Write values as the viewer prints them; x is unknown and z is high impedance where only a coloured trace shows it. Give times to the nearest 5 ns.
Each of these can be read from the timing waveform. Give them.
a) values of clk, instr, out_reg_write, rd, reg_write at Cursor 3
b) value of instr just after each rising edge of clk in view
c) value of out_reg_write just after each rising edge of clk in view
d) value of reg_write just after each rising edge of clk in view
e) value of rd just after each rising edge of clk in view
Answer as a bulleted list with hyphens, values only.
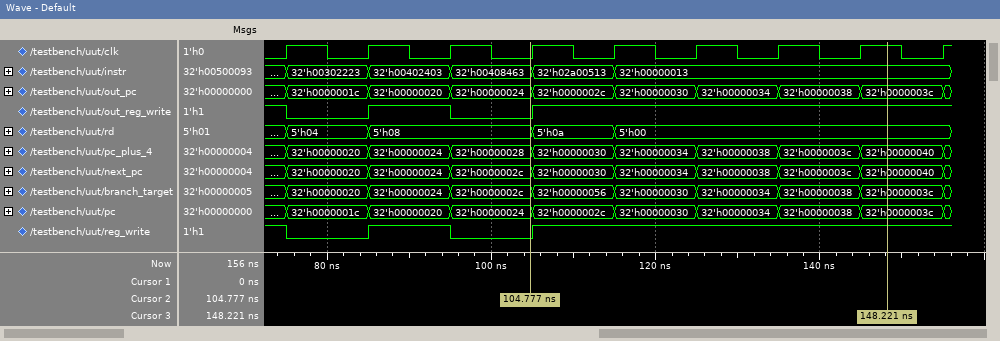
- clk=1, instr=32'h00000013, out_reg_write=1, rd=5'h00, reg_write=1
- 32'h00302223, 32'h00402403, 32'h00408463, 32'h02a00513, 32'h00000013, 32'h00000013, 32'h00000013, 32'h00000013, 32'h00000013
- 0 1 0 1 1 1 1 1 1
- 0 1 0 1 1 1 1 1 1
- 5'h04, 5'h08, 5'h08, 5'h0a, 5'h00, 5'h00, 5'h00, 5'h00, 5'h00
